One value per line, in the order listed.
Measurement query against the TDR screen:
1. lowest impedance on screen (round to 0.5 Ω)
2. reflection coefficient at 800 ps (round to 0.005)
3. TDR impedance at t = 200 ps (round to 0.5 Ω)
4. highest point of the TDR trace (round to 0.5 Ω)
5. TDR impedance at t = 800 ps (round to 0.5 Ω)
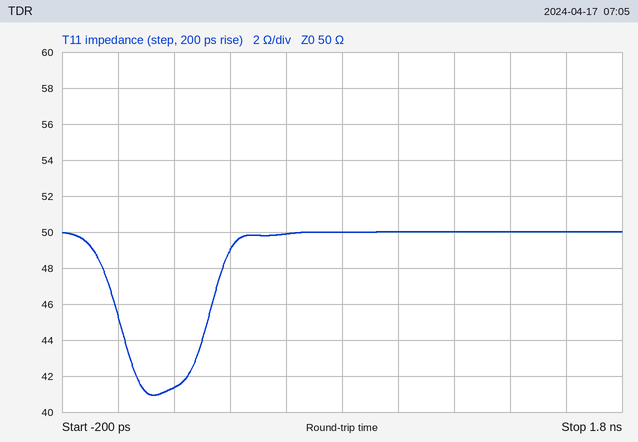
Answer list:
41.0 Ω
0.000
41.5 Ω
50.0 Ω
50.0 Ω
